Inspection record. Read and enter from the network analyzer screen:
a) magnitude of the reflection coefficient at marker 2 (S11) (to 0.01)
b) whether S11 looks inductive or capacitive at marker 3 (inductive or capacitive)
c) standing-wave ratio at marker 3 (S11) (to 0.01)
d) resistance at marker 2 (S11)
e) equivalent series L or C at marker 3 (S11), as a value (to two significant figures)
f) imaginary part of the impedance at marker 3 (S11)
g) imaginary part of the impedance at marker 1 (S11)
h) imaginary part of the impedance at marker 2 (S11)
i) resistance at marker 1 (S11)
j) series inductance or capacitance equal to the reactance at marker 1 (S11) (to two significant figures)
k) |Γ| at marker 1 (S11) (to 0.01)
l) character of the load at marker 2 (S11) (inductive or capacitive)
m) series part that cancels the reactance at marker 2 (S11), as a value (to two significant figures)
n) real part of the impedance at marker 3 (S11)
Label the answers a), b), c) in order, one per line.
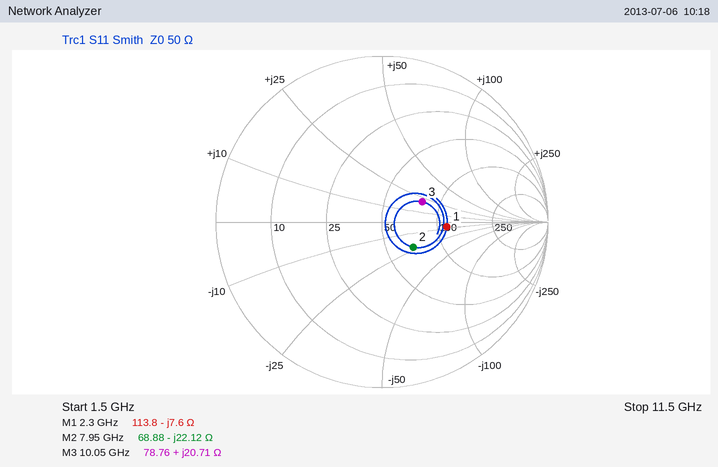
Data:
a) 0.24
b) inductive
c) 1.75
d) 68.88 Ω
e) 330 pH
f) +20.71 Ω
g) -7.6 Ω
h) -22.12 Ω
i) 113.8 Ω
j) 9.1 pF
k) 0.39
l) capacitive
m) 440 pH
n) 78.76 Ω
